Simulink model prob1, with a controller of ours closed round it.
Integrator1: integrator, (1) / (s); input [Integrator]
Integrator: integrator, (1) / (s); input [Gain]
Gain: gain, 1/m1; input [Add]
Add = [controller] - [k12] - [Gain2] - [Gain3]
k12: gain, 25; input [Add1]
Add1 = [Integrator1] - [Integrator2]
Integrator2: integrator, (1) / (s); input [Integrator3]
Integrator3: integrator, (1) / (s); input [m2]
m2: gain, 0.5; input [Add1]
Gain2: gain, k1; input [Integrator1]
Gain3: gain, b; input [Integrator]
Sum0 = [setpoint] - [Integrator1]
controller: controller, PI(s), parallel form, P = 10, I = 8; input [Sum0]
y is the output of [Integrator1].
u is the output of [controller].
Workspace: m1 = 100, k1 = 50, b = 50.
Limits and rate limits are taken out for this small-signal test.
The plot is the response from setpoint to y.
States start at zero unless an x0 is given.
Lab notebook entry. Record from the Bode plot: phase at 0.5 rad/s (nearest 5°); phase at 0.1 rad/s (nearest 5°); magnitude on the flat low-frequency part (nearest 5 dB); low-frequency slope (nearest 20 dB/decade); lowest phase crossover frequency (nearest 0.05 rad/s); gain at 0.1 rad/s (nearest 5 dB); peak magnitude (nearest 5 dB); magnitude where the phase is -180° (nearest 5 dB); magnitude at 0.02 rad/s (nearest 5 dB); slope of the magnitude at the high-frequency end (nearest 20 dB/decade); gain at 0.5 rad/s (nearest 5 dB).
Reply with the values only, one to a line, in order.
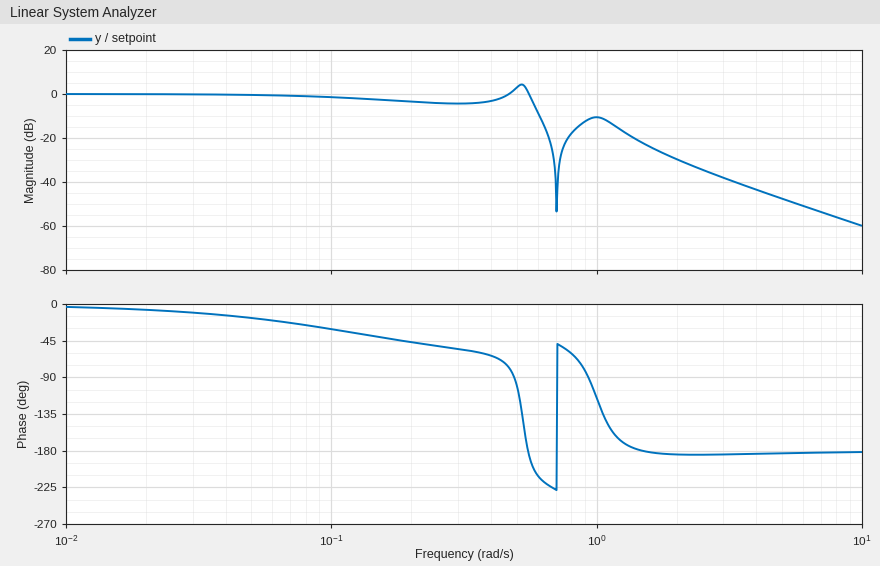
-100°
-30°
0 dB
0 dB/decade
0.55 rad/s
0 dB
5 dB
0 dB
0 dB
-40 dB/decade
5 dB
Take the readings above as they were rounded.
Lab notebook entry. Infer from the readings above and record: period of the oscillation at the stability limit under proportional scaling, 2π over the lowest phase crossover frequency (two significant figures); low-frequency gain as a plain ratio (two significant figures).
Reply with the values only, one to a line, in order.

11 s
1.0
